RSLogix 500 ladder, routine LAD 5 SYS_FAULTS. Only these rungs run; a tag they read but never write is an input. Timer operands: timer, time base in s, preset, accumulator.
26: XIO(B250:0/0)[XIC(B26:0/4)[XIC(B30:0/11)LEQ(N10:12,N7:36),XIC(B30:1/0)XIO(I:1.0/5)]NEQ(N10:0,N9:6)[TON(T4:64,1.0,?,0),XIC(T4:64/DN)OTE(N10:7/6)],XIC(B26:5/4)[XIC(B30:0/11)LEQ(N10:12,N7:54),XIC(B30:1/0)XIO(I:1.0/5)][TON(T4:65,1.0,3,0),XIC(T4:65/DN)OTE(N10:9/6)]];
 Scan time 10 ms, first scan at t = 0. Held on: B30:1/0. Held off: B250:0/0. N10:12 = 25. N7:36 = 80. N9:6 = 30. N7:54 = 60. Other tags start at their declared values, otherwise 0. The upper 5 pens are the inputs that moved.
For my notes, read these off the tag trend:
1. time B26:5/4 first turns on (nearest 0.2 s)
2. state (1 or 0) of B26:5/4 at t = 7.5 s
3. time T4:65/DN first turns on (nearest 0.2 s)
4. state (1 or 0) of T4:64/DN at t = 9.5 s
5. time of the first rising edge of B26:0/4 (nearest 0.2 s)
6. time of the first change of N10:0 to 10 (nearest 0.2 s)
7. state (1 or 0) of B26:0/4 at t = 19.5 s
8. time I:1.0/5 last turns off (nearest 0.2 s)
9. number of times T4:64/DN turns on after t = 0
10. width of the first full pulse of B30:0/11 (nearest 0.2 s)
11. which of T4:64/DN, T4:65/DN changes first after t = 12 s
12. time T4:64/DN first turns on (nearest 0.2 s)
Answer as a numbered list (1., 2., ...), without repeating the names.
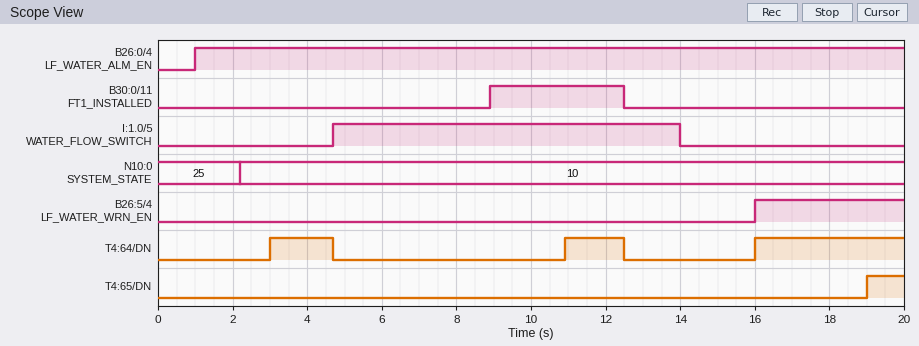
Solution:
1. 16.0 s
2. 0
3. 19.0 s
4. 0
5. 1.0 s
6. 2.2 s
7. 1
8. 14.0 s
9. 3
10. 3.6 s
11. T4:64/DN
12. 3.0 s
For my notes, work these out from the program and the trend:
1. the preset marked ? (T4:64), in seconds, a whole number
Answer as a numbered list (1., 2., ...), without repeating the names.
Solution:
1. 2 s
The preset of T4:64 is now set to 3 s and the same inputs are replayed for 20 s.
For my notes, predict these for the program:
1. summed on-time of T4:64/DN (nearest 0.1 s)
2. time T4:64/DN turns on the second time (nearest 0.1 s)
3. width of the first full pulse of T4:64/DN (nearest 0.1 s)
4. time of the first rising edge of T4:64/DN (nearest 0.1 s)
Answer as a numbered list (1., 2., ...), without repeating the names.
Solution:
1. 4.3 s
2. 11.9 s
3. 0.7 s
4. 4.0 s
